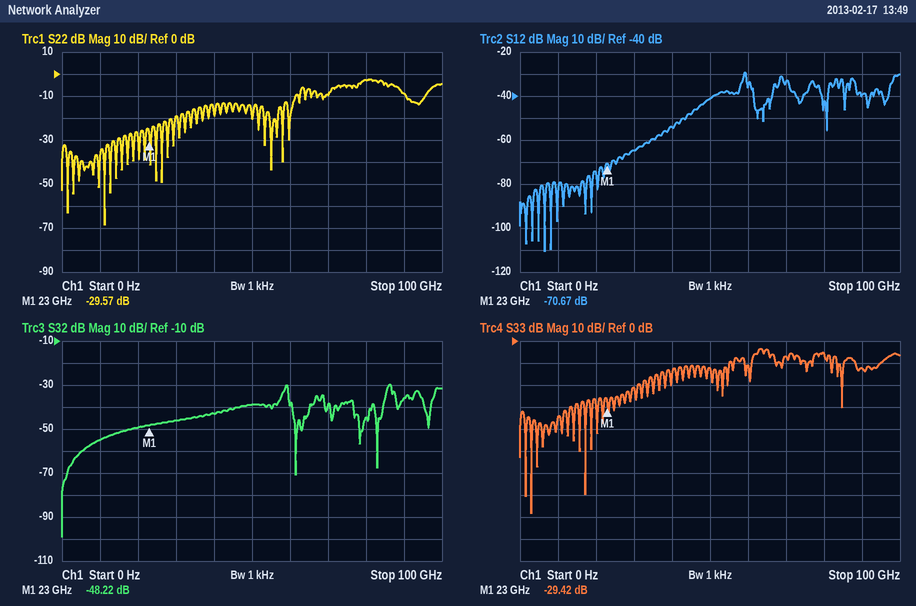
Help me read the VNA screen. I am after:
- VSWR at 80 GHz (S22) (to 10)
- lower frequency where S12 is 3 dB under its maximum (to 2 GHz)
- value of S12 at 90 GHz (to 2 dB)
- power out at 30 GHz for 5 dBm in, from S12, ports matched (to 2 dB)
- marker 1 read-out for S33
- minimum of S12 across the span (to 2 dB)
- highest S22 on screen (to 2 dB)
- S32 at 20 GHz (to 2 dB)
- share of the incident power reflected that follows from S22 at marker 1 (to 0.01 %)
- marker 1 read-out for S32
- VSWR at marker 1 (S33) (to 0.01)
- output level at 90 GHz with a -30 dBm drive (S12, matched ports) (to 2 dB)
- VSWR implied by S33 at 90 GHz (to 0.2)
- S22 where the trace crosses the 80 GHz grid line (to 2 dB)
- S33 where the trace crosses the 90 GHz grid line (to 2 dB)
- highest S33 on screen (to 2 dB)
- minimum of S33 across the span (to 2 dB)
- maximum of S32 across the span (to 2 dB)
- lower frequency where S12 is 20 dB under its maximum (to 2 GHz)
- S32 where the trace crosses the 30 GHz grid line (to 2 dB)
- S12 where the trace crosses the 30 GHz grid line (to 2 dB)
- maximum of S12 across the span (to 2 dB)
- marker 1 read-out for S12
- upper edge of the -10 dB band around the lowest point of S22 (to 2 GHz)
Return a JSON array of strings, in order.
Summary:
["10", "58 GHz", "-40 dB", "-60 dBm", "-29.42 dB", "-110 dB", "-2 dB", "-50 dB", "0.11 %", "-48.22 dB", "1.07", "-70 dBm", "1.6", "-2 dB", "-12 dB", "-4 dB", "-78 dB", "-30 dB", "44 GHz", "-46 dB", "-64 dB", "-30 dB", "-70.67 dB", "62 GHz"]
